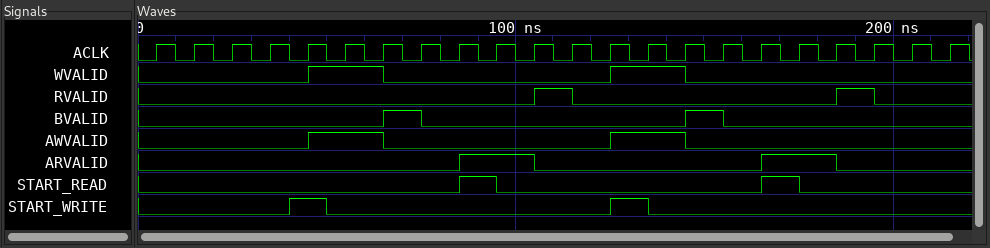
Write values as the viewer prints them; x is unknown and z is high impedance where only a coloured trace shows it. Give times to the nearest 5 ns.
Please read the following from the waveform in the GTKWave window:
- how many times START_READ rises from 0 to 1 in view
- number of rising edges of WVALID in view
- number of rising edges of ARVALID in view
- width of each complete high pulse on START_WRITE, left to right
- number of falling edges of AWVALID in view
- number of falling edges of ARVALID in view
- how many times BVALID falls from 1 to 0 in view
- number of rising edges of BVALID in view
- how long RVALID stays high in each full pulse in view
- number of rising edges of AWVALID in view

2
2
2
10 ns, 10 ns
2
2
2
2
10 ns, 10 ns
2
